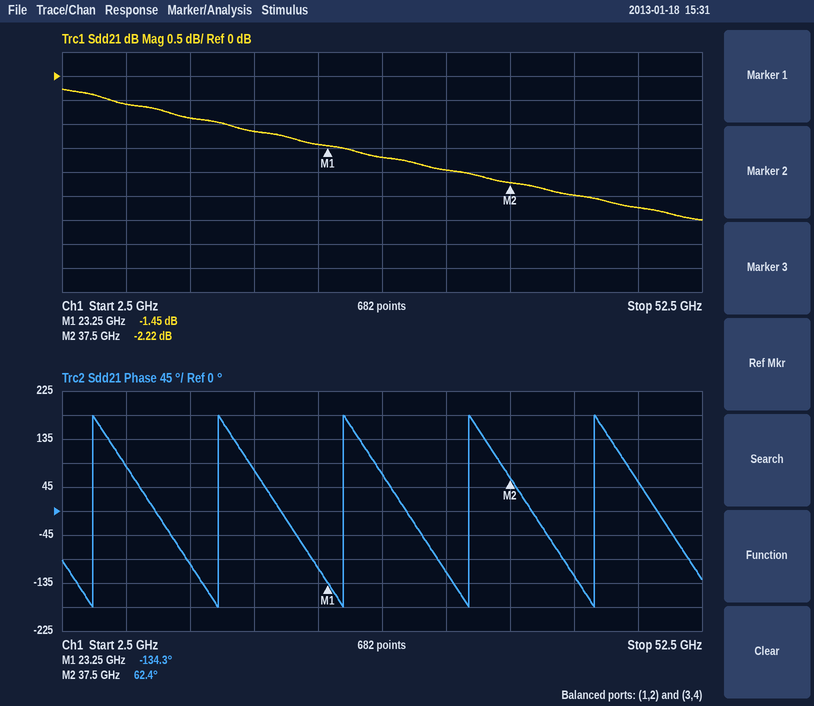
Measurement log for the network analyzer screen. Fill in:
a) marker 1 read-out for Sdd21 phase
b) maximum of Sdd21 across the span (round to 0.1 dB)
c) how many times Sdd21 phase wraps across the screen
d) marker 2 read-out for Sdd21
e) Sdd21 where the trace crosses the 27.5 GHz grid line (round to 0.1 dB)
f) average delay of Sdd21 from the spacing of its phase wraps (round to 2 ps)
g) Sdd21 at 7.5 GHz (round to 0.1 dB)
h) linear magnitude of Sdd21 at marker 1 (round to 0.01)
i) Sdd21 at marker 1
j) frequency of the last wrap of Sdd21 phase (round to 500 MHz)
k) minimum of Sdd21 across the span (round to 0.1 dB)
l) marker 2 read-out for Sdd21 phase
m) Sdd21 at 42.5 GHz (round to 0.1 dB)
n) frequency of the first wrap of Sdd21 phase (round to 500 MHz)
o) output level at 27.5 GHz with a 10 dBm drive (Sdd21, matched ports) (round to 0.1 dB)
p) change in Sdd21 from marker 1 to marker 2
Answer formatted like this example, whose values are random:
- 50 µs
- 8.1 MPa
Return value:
- -134.3°
- -0.3 dB
- 5
- -2.22 dB
- -1.7 dB
- 102 ps
- -0.6 dB
- 0.85
- -1.45 dB
- 44.0 GHz
- -3.0 dB
- 62.4°
- -2.5 dB
- 5.0 GHz
- 8.3 dBm
- -0.77 dB
